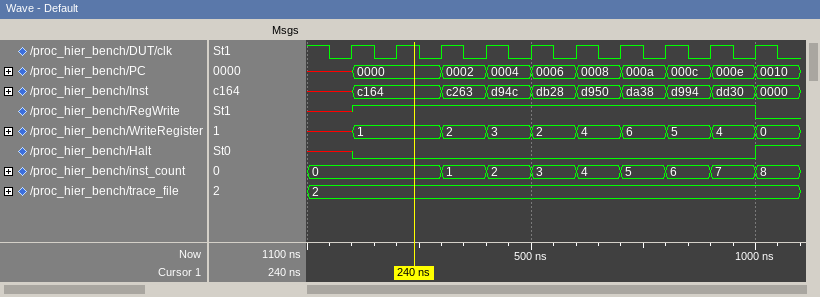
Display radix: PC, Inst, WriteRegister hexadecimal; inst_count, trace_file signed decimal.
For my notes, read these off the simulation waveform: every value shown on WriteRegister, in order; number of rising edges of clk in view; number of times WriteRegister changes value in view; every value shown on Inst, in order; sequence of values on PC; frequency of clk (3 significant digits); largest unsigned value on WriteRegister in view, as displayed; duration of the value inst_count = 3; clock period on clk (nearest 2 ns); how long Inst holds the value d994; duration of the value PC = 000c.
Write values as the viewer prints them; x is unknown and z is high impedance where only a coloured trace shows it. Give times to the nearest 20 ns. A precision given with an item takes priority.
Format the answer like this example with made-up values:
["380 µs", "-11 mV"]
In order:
["x, 1, 2, 3, 2, 4, 6, 5, 4, 0", "10", "9", "x, c164, c263, d94c, db28, d950, da38, d994, dd30, 0000", "x, 0000, 0002, 0004, 0006, 0008, 000a, 000c, 000e, 0010", "10.0 MHz", "6", "100 ns", "100 ns", "100 ns", "100 ns"]
